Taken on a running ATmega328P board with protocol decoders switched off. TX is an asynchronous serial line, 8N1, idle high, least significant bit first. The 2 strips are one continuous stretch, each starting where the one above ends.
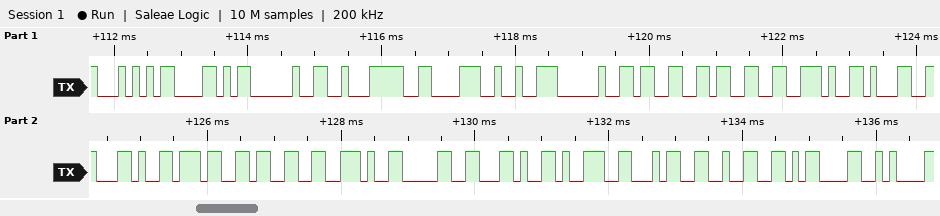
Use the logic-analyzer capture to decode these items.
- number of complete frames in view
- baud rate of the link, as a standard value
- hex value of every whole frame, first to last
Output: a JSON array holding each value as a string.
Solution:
["22", "9600 baud", "54 58 20 E2 86 92 20 33 33 2E 31 2C 37 33 2E 30 2C 39 34 32 0D 0A"]
